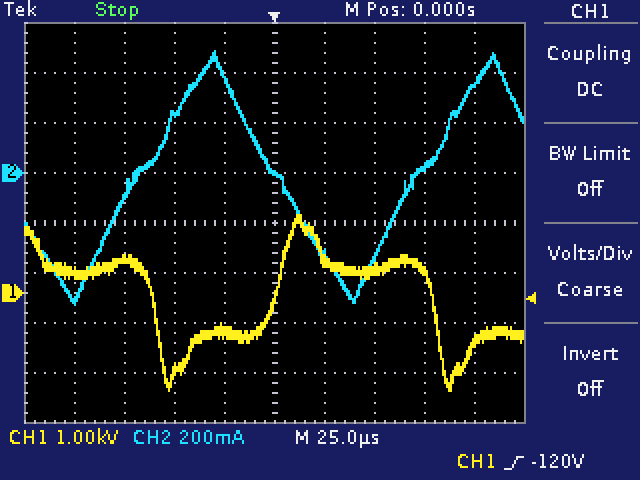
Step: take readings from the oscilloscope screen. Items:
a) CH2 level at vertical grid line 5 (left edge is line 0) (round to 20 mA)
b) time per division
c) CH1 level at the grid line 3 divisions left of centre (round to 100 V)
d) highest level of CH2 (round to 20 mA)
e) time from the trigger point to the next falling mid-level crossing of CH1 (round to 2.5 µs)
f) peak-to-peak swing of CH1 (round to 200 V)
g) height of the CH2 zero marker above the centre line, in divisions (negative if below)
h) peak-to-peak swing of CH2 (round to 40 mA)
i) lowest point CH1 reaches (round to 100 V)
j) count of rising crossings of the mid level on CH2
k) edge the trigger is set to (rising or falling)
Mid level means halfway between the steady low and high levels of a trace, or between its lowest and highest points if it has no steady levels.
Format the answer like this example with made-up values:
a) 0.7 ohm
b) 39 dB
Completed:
a) 0 mA
b) 25 µs
c) 700 V
d) 480 mA
e) 80.0 µs
f) 3.6 kV
g) +1.0 div
h) 1.00 A
i) -2.0 kV
j) 2
k) rising
